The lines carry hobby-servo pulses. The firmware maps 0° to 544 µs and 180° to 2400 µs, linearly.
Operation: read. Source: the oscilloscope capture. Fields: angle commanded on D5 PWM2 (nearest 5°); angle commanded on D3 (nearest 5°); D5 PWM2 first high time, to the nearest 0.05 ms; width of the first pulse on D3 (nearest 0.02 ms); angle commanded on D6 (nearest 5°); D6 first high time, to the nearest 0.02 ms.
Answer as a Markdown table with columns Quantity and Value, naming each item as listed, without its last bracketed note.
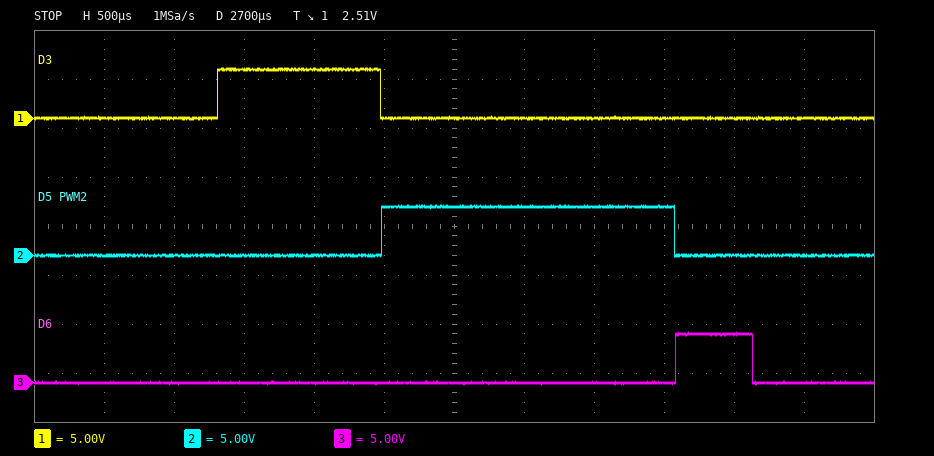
| Quantity | Value |
|---|---|
| angle commanded on D5 PWM2 | 150° |
| angle commanded on D3 | 60° |
| D5 PWM2 first high time, to the nearest 0.05 ms | 2.10 ms |
| width of the first pulse on D3 | 1.16 ms |
| angle commanded on D6 | 0° |
| D6 first high time, to the nearest 0.02 ms | 0.54 ms |
